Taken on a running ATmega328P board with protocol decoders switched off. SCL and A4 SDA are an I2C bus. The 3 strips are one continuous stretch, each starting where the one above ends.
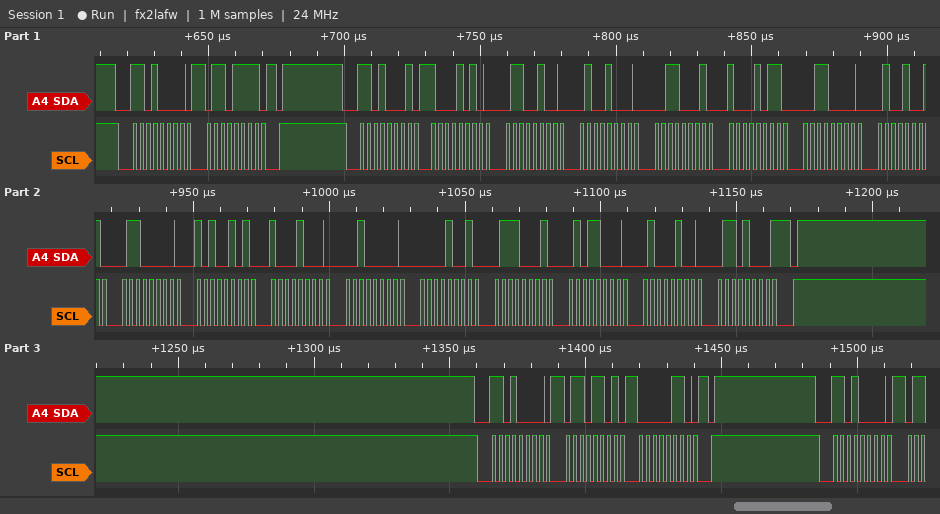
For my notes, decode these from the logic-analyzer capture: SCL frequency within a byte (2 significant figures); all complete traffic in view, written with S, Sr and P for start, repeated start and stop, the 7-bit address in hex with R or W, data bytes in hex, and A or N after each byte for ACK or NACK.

400 kHz
S 68W A 6F A P S 68R A 8A A 64 A 48 A 31 A 8B A 30 A 49 A 60 A A5 A 88 A 20 A 09 A 71 A 58 A 44 A 68 N P S 68W A 6D A 06 A P S 68W A
